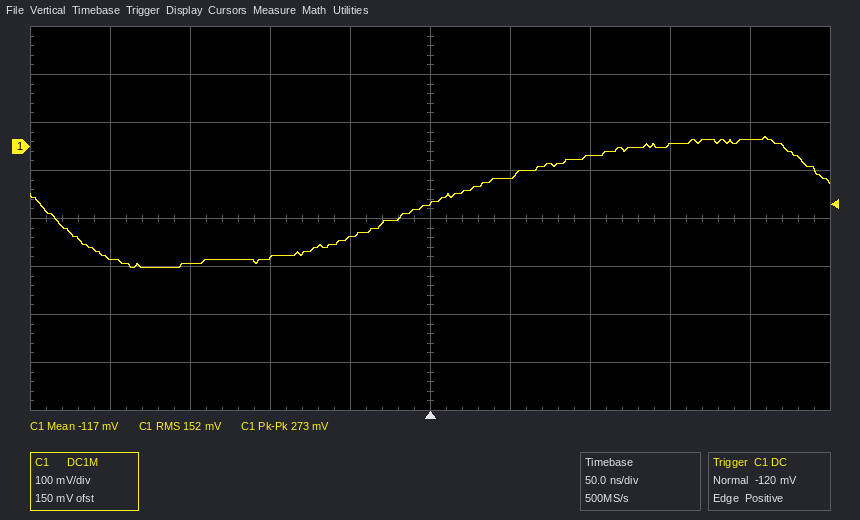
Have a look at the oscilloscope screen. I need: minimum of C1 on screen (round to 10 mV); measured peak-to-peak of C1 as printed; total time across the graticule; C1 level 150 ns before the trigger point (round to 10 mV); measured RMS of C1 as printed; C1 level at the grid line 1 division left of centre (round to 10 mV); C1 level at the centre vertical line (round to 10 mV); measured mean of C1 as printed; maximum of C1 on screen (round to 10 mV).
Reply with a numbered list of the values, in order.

1. -250 mV
2. 273 mV
3. 500 ns
4. -240 mV
5. 152 mV
6. -190 mV
7. -120 mV
8. -117 mV
9. 20 mV
